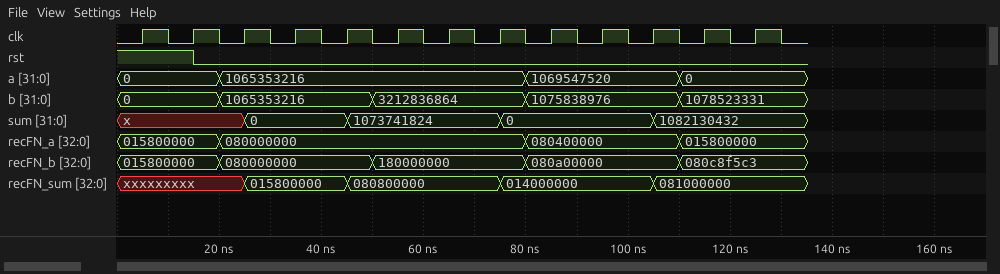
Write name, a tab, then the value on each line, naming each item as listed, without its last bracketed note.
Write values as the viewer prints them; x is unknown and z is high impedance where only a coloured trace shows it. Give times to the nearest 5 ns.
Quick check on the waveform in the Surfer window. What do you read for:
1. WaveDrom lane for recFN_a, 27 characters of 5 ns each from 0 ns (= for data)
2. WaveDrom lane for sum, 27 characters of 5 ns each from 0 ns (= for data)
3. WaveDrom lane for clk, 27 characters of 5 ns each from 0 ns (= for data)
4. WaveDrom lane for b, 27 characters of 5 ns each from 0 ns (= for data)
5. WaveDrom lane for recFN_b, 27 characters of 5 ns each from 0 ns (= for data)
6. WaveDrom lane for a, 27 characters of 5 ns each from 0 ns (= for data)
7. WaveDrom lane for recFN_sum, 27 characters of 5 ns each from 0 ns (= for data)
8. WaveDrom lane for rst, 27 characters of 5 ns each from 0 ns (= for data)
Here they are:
WaveDrom lane for recFN_a, 27 characters of 5 ns each from 0 ns	{name: 'recFN_a', wave: '=...=...........=.....=....', data: '015800000 080000000 080400000 015800000'}
WaveDrom lane for sum, 27 characters of 5 ns each from 0 ns	{name: 'sum', wave: 'x....=...=.....=.....=.....', data: '0 1073741824 0 1082130432'}
WaveDrom lane for clk, 27 characters of 5 ns each from 0 ns	{name: 'clk', wave: '010101010101010101010101010'}
WaveDrom lane for b, 27 characters of 5 ns each from 0 ns	{name: 'b', wave: '=...=.....=.....=.....=....', data: '0 1065353216 3212836864 1075838976 1078523331'}
WaveDrom lane for recFN_b, 27 characters of 5 ns each from 0 ns	{name: 'recFN_b', wave: '=...=.....=.....=.....=....', data: '015800000 080000000 180000000 080a00000 080c8f5c3'}
WaveDrom lane for a, 27 characters of 5 ns each from 0 ns	{name: 'a', wave: '=...=...........=.....=....', data: '0 1065353216 1069547520 0'}
WaveDrom lane for recFN_sum, 27 characters of 5 ns each from 0 ns	{name: 'recFN_sum', wave: 'x....=...=.....=.....=.....', data: '015800000 080800000 014000000 081000000'}
WaveDrom lane for rst, 27 characters of 5 ns each from 0 ns	{name: 'rst', wave: '1..0.......................'}
